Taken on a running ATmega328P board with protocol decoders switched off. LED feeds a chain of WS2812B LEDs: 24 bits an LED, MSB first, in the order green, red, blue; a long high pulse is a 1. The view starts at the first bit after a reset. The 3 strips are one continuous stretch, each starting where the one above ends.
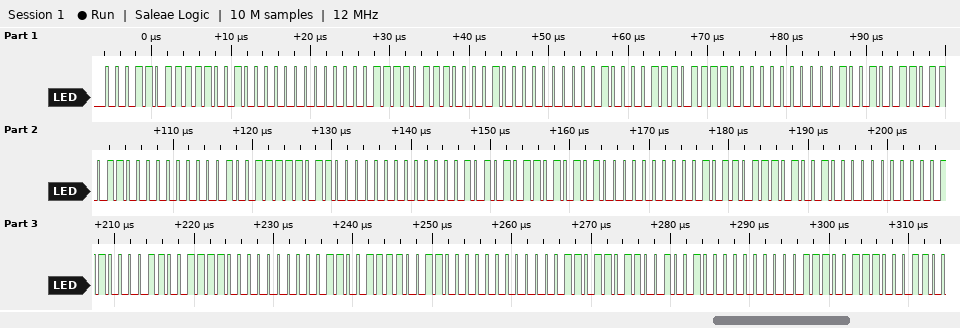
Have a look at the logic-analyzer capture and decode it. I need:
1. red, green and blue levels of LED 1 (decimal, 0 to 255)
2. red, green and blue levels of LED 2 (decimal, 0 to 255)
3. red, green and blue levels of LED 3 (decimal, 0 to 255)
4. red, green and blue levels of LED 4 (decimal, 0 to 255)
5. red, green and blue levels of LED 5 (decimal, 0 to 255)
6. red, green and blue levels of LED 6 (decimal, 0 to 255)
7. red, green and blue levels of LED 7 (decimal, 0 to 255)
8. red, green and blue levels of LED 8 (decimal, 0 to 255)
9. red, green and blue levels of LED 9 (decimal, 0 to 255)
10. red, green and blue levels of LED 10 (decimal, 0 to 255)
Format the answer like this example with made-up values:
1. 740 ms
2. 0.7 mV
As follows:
1. 228, 27, 0
2. 225, 30, 0
3. 222, 33, 0
4. 219, 36, 0
5. 216, 39, 0
6. 213, 42, 0
7. 210, 45, 0
8. 207, 48, 0
9. 204, 51, 0
10. 201, 54, 0
